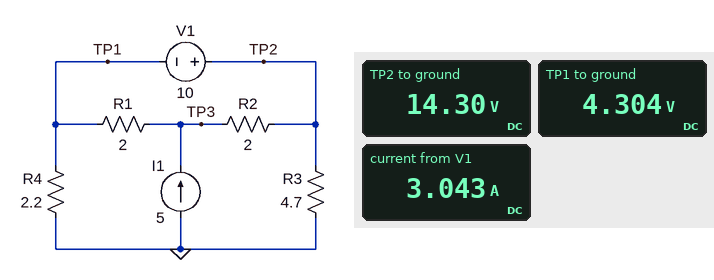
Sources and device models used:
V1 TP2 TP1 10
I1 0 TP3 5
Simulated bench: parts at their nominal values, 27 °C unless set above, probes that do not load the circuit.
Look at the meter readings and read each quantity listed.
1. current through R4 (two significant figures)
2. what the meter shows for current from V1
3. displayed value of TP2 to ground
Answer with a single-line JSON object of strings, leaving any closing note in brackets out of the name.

{"current through R4": "2.0 A", "what the meter shows for current from V1": "3.043 A", "displayed value of TP2 to ground": "14.30 V"}
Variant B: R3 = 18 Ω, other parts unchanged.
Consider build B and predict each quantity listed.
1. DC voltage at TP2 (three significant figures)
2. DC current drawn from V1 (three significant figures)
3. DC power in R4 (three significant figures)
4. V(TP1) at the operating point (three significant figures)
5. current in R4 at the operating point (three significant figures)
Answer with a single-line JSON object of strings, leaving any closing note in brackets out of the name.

{"DC voltage at TP2": "18.7 V", "DC current drawn from V1": "1.04 A", "DC power in R4": "34.5 W", "V(TP1) at the operating point": "8.71 V", "current in R4 at the operating point": "3.96 A"}
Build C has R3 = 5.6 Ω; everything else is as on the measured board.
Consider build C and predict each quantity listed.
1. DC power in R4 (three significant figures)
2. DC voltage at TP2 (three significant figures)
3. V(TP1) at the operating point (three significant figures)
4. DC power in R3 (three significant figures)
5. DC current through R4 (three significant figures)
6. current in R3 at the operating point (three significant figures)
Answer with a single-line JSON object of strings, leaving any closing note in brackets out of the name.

{"DC power in R4": "11.7 W", "DC voltage at TP2": "15.1 V", "V(TP1) at the operating point": "5.08 V", "DC power in R3": "40.6 W", "DC current through R4": "2.31 A", "current in R3 at the operating point": "2.69 A"}
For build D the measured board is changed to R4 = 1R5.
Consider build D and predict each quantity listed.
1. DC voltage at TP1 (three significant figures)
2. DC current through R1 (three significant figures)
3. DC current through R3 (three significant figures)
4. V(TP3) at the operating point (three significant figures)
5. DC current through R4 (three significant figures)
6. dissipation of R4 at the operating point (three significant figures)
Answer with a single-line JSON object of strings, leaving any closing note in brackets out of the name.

{"DC voltage at TP1": "3.27 V", "DC current through R1": "5.00 A", "DC current through R3": "2.82 A", "V(TP3) at the operating point": "13.3 V", "DC current through R4": "2.18 A", "dissipation of R4 at the operating point": "7.11 W"}
